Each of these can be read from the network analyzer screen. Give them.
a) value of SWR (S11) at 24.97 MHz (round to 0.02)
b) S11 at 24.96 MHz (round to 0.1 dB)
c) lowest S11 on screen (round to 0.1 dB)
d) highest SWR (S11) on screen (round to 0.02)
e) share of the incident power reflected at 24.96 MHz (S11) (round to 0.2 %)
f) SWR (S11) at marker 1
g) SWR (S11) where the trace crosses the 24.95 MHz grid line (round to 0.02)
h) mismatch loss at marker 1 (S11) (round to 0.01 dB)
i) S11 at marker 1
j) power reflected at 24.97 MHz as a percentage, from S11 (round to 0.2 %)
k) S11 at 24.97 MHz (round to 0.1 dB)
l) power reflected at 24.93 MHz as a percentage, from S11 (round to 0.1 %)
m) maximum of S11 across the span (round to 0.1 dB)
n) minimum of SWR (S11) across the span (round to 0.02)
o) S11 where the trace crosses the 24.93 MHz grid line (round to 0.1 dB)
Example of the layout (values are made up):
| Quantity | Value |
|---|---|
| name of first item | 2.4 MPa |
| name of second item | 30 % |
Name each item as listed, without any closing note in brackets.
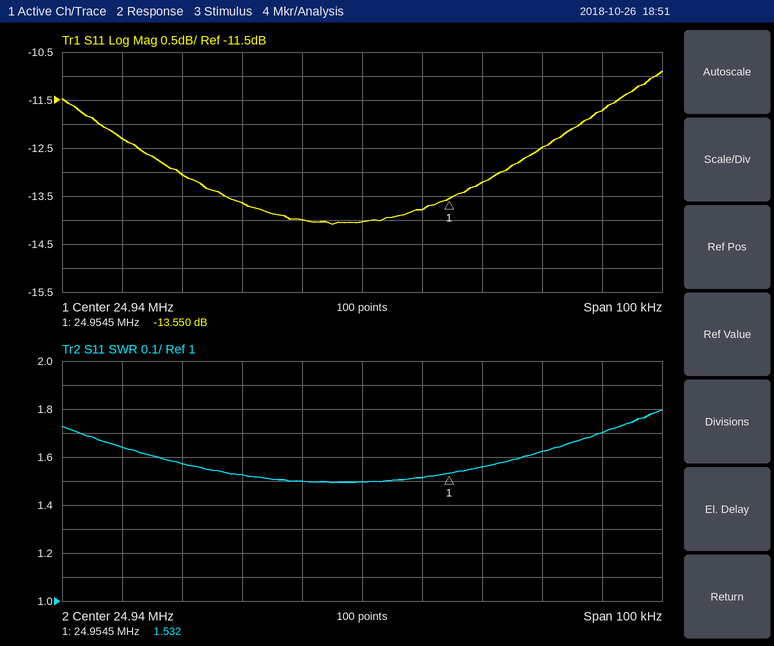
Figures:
| Quantity | Value |
|---|---|
| value of SWR (S11) at 24.97 MHz | 1.62 |
| S11 at 24.96 MHz | -13.2 dB |
| lowest S11 on screen | -14.1 dB |
| highest SWR (S11) on screen | 1.80 |
| share of the incident power reflected at 24.96 MHz (S11) | 4.8 % |
| SWR (S11) at marker 1 | 1.532 |
| SWR (S11) where the trace crosses the 24.95 MHz grid line | 1.52 |
| mismatch loss at marker 1 (S11) | 0.20 dB |
| S11 at marker 1 | -13.550 dB |
| power reflected at 24.97 MHz as a percentage, from S11 | 5.6 % |
| S11 at 24.97 MHz | -12.5 dB |
| power reflected at 24.93 MHz as a percentage, from S11 | 4.0 % |
| maximum of S11 across the span | -10.9 dB |
| minimum of SWR (S11) across the span | 1.50 |
| S11 where the trace crosses the 24.93 MHz grid line | -14.0 dB |
